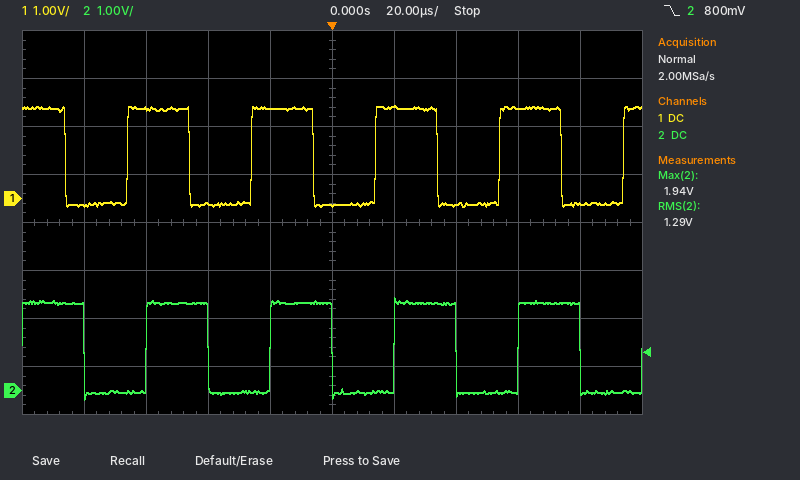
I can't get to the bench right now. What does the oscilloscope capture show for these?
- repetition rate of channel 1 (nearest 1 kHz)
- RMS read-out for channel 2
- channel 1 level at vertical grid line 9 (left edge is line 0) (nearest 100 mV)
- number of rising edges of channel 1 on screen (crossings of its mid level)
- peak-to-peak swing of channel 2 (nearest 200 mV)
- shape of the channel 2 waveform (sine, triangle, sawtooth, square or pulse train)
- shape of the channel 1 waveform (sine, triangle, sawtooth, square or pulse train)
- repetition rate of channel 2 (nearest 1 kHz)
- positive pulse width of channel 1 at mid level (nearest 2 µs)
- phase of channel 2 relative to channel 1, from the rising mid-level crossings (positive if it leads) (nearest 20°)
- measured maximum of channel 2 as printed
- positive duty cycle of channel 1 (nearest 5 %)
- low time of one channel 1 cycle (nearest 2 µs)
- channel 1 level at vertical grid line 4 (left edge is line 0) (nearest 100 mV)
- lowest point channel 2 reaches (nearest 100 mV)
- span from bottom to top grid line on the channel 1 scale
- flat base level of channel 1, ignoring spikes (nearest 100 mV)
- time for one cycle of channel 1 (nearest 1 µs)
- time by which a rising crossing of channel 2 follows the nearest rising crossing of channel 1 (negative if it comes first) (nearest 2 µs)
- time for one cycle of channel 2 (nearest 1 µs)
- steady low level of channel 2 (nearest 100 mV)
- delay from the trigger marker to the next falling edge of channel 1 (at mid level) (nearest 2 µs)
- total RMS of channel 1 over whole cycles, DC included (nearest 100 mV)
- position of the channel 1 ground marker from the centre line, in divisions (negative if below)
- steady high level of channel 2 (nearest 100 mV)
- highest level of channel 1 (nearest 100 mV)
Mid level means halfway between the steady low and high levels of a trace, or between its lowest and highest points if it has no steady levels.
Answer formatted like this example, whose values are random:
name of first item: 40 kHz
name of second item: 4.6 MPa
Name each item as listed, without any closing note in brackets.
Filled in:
repetition rate of channel 1: 25 kHz
RMS read-out for channel 2: 1.29 V
channel 1 level at vertical grid line 9 (left edge is line 0): -100 mV
number of rising edges of channel 1 on screen: 5
peak-to-peak swing of channel 2: 2.2 V
shape of the channel 2 waveform: square
shape of the channel 1 waveform: square
repetition rate of channel 2: 25 kHz
positive pulse width of channel 1 at mid level: 20 µs
phase of channel 2 relative to channel 1, from the rising mid-level crossings (positive if it leads): -60°
measured maximum of channel 2 as printed: 1.94 V
positive duty cycle of channel 1: 50 %
low time of one channel 1 cycle: 20 µs
channel 1 level at vertical grid line 4 (left edge is line 0): 1.9 V
lowest point channel 2 reaches: -200 mV
span from bottom to top grid line on the channel 1 scale: 8 V
flat base level of channel 1, ignoring spikes: -100 mV
time for one cycle of channel 1: 40 µs
time by which a rising crossing of channel 2 follows the nearest rising crossing of channel 1 (negative if it comes first): +6 µs
time for one cycle of channel 2: 40 µs
steady low level of channel 2: 0.0 V
delay from the trigger marker to the next falling edge of channel 1 (at mid level): 34 µs
total RMS of channel 1 over whole cycles, DC included: 1.3 V
position of the channel 1 ground marker from the centre line, in divisions: +0.5 div
steady high level of channel 2: 1.8 V
highest level of channel 1: 1.9 V
